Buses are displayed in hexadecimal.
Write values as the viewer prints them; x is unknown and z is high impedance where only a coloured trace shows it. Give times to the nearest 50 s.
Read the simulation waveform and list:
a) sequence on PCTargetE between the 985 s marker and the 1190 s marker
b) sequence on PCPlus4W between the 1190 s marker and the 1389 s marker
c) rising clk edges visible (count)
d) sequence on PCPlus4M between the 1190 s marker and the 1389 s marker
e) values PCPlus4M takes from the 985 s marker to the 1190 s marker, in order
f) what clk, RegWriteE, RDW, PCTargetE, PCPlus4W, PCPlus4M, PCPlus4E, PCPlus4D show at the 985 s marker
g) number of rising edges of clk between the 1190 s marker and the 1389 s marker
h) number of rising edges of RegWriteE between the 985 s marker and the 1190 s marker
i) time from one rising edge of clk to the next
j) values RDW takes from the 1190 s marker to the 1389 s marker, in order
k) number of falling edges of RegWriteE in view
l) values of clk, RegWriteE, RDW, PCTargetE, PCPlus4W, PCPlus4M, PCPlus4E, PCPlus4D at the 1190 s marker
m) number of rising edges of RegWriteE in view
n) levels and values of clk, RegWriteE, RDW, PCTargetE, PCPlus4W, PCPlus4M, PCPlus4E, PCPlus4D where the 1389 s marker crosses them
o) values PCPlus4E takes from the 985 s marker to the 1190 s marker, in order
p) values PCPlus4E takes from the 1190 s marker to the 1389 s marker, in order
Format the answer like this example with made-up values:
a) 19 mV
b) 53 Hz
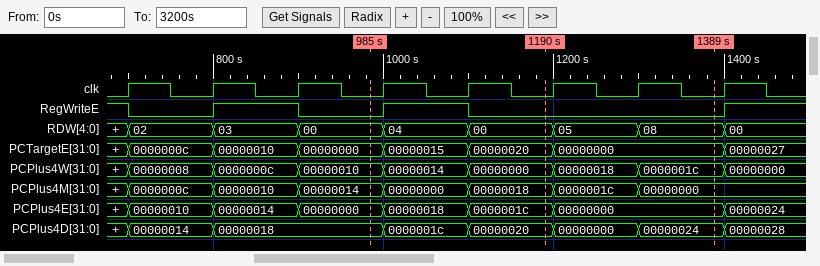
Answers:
a) 00000000, 00000015, 00000020
b) 00000000, 00000018, 0000001c
c) 8
d) 00000018, 0000001c, 00000000
e) 00000014, 00000000, 00000018
f) clk=0, RegWriteE=0, RDW=00, PCTargetE=00000000, PCPlus4W=00000010, PCPlus4M=00000014, PCPlus4E=00000000, PCPlus4D=00000018
g) 2
h) 1
i) 100 s
j) 00, 05, 08
k) 3
l) clk=0, RegWriteE=0, RDW=00, PCTargetE=00000020, PCPlus4W=00000000, PCPlus4M=00000018, PCPlus4E=0000001c, PCPlus4D=00000020
m) 3
n) clk=0, RegWriteE=0, RDW=08, PCTargetE=00000000, PCPlus4W=0000001c, PCPlus4M=00000000, PCPlus4E=00000000, PCPlus4D=00000024
o) 00000000, 00000018, 0000001c
p) 0000001c, 00000000
